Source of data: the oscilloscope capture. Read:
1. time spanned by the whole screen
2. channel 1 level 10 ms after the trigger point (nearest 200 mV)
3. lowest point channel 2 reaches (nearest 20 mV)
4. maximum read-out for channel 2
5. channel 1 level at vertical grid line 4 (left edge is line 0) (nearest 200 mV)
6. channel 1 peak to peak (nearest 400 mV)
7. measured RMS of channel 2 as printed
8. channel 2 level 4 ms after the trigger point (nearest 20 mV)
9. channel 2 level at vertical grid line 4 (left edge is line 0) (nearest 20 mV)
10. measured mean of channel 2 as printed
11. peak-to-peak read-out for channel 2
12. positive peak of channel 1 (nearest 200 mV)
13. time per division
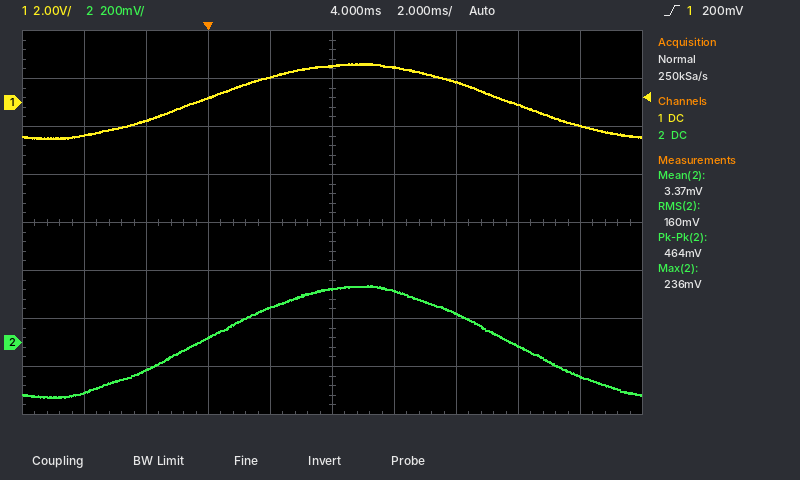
20 ms
0.0 V
-220 mV
236 mV
1.0 V
3.2 V
160 mV
220 mV
140 mV
3.37 mV
464 mV
1.6 V
2 ms
